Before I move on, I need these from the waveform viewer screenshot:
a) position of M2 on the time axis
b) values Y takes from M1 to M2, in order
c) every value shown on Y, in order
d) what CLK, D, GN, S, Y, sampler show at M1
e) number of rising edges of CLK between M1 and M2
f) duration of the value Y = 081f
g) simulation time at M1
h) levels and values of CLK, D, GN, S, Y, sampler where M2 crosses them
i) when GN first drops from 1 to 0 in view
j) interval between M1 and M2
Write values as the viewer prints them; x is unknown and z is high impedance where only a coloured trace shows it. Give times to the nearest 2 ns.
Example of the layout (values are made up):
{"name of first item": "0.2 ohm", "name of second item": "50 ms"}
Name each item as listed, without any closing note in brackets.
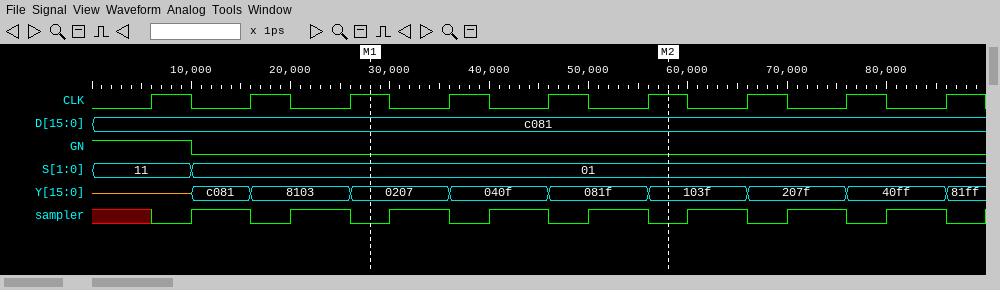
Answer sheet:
{"position of M2 on the time axis": "58 ns", "values Y takes from M1 to M2, in order": "0207, 040f, 081f, 103f", "every value shown on Y, in order": "z, c081, 8103, 0207, 040f, 081f, 103f, 207f, 40ff, 81ff", "what CLK, D, GN, S, Y, sampler show at M1": "CLK=1, D=c081, GN=0, S=01, Y=0207, sampler=0", "number of rising edges of CLK between M1 and M2": "3", "duration of the value Y = 081f": "10 ns", "simulation time at M1": "28 ns", "levels and values of CLK, D, GN, S, Y, sampler where M2 crosses them": "CLK=1, D=c081, GN=0, S=01, Y=103f, sampler=0", "when GN first drops from 1 to 0 in view": "10 ns", "interval between M1 and M2": "30 ns"}
